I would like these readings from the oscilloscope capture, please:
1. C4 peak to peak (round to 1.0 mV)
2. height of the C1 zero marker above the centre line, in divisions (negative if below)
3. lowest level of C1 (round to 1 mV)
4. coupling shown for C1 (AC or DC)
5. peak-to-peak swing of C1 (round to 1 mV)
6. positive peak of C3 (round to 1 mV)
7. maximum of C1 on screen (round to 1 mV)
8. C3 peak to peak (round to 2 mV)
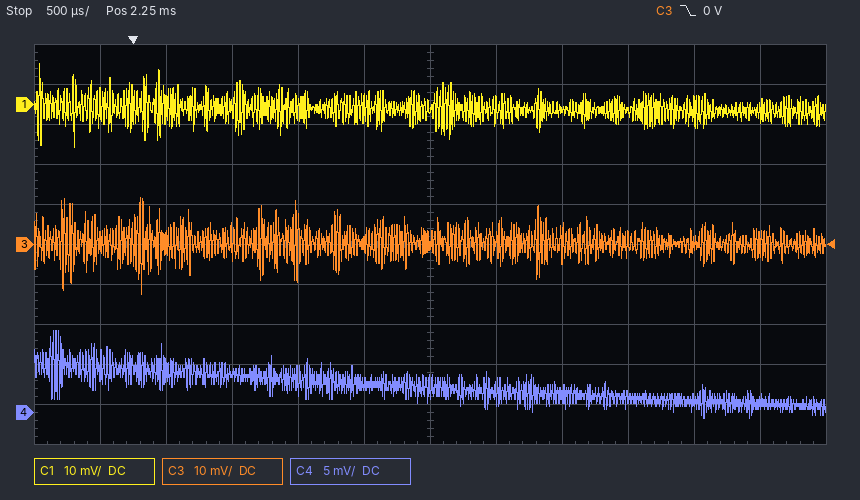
11.0 mV
+3.5 div
-11 mV
DC
21 mV
12 mV
10 mV
24 mV
